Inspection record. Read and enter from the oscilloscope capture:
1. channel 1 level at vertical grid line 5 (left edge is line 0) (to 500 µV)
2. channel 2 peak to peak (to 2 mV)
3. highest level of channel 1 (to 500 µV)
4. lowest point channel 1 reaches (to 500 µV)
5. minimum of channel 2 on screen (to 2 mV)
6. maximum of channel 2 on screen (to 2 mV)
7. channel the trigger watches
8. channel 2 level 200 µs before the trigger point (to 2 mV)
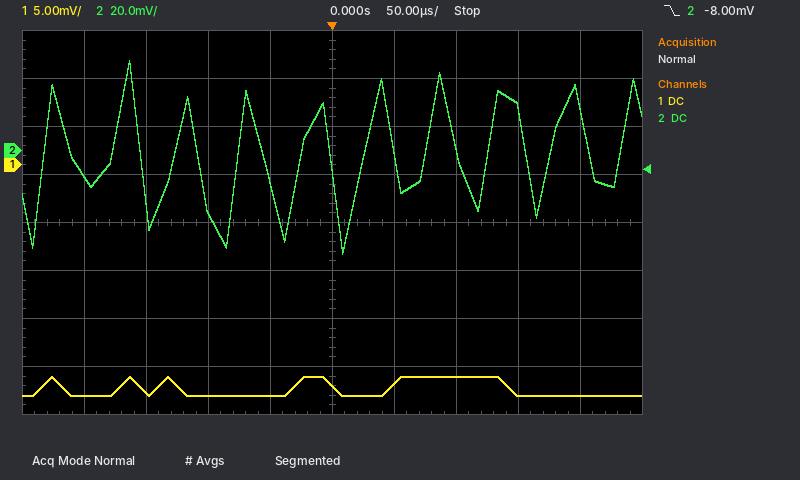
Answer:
-23.0 mV
80 mV
-22.0 mV
-24.0 mV
-42 mV
38 mV
channel 2
-10 mV
